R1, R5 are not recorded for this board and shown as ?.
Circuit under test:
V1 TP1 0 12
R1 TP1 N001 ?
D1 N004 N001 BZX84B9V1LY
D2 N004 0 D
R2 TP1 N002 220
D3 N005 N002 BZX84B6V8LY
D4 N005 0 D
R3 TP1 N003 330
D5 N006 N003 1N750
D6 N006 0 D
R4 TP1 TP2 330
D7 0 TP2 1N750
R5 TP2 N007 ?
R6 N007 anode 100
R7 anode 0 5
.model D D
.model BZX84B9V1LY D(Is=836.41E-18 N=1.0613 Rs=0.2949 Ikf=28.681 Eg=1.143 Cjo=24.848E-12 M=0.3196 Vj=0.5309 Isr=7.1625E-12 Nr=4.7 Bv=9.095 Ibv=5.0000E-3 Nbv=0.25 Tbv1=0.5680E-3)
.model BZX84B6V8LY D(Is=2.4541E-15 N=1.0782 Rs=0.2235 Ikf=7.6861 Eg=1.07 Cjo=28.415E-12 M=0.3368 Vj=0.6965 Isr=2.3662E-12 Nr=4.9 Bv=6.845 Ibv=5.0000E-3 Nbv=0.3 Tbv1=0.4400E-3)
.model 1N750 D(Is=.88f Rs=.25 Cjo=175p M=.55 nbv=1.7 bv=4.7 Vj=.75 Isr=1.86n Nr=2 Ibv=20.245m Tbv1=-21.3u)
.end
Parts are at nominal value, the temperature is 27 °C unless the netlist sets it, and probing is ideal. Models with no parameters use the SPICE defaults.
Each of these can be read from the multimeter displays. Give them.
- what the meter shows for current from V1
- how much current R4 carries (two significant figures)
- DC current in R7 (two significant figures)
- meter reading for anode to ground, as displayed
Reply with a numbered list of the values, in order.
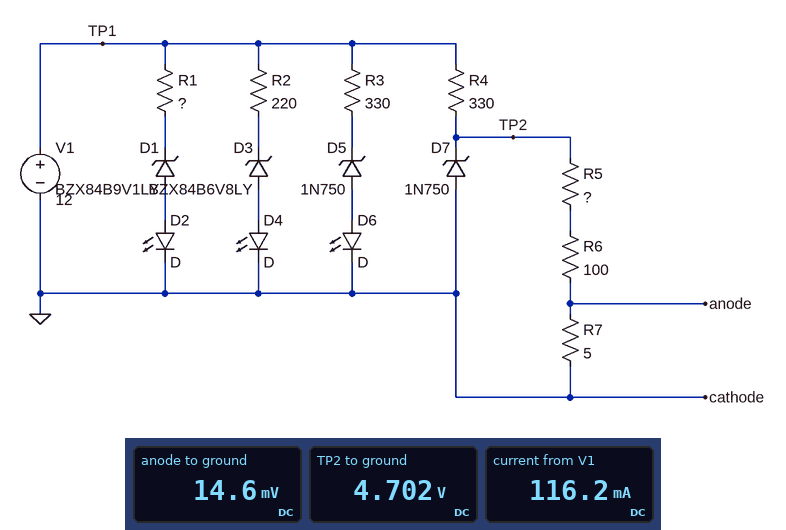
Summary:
1. 116.2 mA
2. 22 mA
3. 2.9 mA
4. 14.6 mV
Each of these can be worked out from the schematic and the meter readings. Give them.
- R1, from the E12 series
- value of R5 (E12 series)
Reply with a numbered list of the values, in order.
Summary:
1. 39 Ω
2. 1.5 kΩ
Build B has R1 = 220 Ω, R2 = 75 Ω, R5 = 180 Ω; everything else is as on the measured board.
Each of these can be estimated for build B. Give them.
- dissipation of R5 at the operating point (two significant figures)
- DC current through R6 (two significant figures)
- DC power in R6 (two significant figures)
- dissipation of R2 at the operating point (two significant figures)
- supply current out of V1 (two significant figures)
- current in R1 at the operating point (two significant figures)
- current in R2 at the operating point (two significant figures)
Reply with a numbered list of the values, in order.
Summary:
1. 48 mW
2. 16 mA
3. 27 mW
4. 250 mW
5. 110 mA
6. 9.9 mA
7. 58 mA
